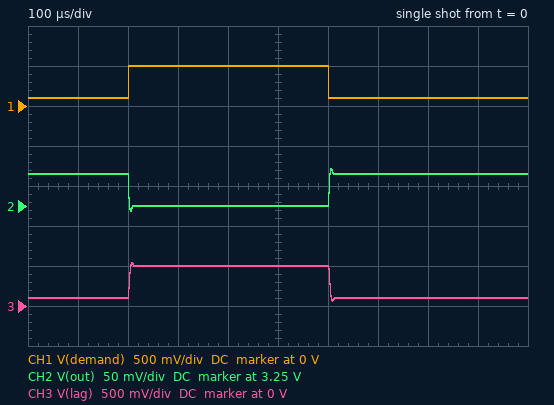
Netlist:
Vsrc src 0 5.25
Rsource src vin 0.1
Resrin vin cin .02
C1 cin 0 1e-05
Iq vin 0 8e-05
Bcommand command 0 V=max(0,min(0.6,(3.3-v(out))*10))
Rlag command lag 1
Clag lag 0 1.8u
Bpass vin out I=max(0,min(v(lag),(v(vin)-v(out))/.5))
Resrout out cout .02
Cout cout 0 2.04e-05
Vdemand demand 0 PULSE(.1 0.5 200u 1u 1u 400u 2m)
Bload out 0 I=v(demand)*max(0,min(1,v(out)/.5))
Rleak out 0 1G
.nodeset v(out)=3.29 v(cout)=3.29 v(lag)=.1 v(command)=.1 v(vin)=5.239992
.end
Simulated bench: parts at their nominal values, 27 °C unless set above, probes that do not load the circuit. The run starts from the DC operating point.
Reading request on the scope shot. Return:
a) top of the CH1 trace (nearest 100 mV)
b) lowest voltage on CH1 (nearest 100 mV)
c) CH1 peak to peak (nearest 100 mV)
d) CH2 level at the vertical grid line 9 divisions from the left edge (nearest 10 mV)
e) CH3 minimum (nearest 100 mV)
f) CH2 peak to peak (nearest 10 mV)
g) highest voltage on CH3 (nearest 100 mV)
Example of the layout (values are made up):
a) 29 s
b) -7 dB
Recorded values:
a) 500 mV
b) 100 mV
c) 400 mV
d) 3.29 V
e) 100 mV
f) 50 mV
g) 500 mV
